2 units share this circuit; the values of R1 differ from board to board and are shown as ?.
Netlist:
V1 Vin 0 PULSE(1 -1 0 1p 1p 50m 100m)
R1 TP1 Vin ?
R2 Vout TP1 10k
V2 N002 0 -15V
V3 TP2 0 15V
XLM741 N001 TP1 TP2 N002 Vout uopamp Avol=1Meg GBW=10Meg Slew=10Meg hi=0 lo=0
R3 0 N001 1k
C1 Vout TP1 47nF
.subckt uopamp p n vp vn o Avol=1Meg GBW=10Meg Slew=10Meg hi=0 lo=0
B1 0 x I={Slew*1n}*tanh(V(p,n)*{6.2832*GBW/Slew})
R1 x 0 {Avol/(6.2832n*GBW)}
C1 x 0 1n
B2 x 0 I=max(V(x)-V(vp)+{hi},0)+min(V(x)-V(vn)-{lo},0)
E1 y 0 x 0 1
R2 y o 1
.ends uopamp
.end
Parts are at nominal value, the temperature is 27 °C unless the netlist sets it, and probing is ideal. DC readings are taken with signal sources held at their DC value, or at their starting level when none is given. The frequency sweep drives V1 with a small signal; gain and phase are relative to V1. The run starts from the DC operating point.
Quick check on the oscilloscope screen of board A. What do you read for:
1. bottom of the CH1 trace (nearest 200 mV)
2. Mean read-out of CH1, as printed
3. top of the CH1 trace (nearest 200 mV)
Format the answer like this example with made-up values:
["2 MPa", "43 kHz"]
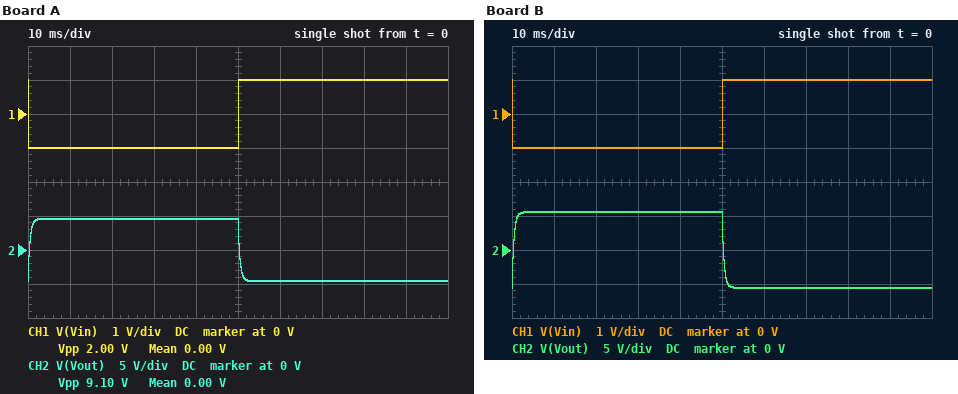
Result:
["-1.0 V", "0.00 V", "1.0 V"]
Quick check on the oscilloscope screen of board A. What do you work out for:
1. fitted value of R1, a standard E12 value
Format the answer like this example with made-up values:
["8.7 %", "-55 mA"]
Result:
["2.2 kΩ"]
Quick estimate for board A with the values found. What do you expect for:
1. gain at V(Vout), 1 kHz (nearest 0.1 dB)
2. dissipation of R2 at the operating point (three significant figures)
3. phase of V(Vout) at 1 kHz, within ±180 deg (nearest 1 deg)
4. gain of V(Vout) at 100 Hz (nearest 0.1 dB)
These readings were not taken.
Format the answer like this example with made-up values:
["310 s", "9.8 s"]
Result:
["3.3 dB", "2.07 mW", "109 deg", "12.8 dB"]
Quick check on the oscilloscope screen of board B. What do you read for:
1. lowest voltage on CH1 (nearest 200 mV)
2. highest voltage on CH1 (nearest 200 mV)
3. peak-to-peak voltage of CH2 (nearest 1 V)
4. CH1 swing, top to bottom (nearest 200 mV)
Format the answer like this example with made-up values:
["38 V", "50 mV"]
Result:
["-1.0 V", "1.0 V", "11 V", "2.0 V"]
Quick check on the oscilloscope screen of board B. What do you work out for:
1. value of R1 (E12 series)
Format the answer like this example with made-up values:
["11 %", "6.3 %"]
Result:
["1.8 kΩ"]
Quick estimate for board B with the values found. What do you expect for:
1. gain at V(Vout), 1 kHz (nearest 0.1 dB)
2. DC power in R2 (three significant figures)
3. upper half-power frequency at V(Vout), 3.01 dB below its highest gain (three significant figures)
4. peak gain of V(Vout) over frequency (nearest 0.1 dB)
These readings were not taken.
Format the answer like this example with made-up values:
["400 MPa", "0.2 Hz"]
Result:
["5.0 dB", "3.09 mW", "339 Hz", "14.9 dB"]
